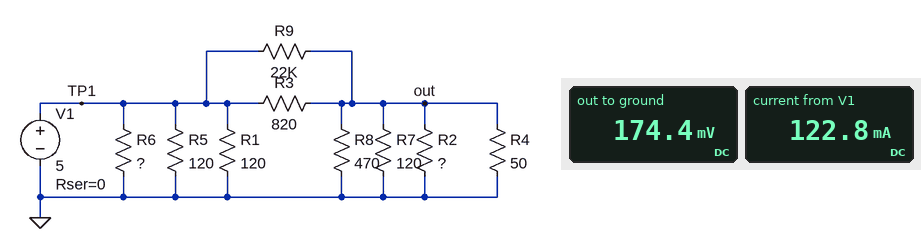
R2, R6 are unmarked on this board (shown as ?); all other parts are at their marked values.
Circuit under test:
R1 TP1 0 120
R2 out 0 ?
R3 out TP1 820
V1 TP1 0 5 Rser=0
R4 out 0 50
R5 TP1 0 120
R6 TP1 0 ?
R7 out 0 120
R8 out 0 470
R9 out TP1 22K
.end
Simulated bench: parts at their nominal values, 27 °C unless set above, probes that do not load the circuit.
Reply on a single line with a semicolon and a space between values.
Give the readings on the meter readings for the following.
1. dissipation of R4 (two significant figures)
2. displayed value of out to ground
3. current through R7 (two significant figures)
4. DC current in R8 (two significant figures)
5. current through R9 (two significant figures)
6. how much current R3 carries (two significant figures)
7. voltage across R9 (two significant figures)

610 µW; 174.4 mV; 1.5 mA; 370 µA; 220 µA; 5.9 mA; 4.8 V
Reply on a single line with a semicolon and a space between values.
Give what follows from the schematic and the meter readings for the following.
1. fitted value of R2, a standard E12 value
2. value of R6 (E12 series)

220 Ω; 150 Ω
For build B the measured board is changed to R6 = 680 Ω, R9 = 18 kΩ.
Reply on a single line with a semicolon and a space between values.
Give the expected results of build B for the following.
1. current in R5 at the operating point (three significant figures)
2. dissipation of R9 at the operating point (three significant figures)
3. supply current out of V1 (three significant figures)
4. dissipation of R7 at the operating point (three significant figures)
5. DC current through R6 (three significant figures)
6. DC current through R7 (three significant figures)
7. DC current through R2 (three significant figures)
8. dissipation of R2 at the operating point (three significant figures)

41.7 mA; 1.29 mW; 96.8 mA; 257 µW; 7.35 mA; 1.46 mA; 799 µA; 140 µW
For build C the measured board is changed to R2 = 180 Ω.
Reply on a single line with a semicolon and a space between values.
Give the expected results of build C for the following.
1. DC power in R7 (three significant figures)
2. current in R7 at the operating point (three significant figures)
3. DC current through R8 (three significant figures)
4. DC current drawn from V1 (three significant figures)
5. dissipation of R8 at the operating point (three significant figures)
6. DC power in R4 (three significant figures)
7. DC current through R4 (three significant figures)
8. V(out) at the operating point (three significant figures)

240 µW; 1.41 mA; 361 µA; 123 mA; 61.2 µW; 576 µW; 3.39 mA; 170 mV
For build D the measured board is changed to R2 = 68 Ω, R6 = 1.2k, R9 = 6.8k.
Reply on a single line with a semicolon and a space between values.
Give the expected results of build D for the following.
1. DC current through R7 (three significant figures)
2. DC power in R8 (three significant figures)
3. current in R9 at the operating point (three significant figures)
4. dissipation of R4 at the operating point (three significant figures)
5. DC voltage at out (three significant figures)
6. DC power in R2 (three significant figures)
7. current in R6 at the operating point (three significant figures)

1.22 mA; 45.9 µW; 714 µA; 431 µW; 147 mV; 317 µW; 4.17 mA
